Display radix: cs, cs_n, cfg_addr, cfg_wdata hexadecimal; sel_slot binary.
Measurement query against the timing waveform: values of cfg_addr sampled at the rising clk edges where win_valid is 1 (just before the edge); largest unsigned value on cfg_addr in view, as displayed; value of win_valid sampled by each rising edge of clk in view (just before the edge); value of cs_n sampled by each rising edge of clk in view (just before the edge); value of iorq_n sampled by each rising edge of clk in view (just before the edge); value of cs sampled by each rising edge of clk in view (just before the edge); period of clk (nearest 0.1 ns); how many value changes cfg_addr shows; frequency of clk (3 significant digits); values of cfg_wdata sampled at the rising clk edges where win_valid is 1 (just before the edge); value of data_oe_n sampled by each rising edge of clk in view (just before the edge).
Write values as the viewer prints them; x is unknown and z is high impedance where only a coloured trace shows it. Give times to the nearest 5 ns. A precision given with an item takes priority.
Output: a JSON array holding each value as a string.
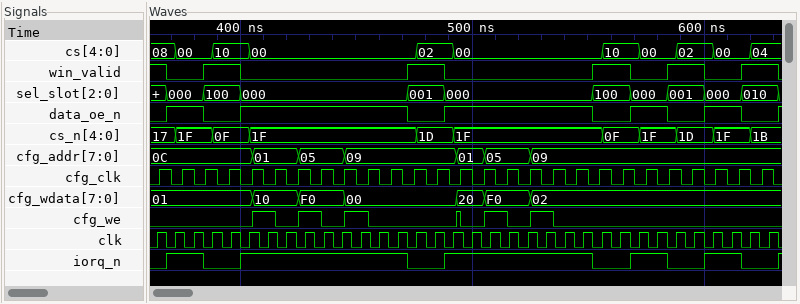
["0C, 0C, 0C, 09, 09, 09, 09, 09, 09, 09, 09", "0C", "1 0 0 1 1 0 0 0 0 0 0 0 0 0 1 1 0 0 0 0 0 0 0 0 1 1 0 0 1 1 0 0 1 1", "17, 17, 1F, 1F, 0F, 0F, 1F, 1F, 1F, 1F, 1F, 1F, 1F, 1F, 1F, 1D, 1D, 1F, 1F, 1F, 1F, 1F, 1F, 1F, 1F, 0F, 0F, 1F, 1F, 1D, 1D, 1F, 1F, 1B", "0 1 1 0 0 1 1 1 1 1 1 1 1 1 0 0 1 1 1 1 1 1 1 1 0 0 1 1 0 0 1 1 0 0", "08, 08, 00, 00, 10, 10, 00, 00, 00, 00, 00, 00, 00, 00, 00, 02, 02, 00, 00, 00, 00, 00, 00, 00, 00, 10, 10, 00, 00, 02, 02, 00, 00, 04", "8 ns", "6", "125 MHz", "01, 01, 01, 00, 00, 02, 02, 02, 02, 02, 02", "0 1 1 0 0 1 1 1 1 1 1 1 1 1 0 0 1 1 1 1 1 1 1 1 0 0 1 1 0 0 1 1 0 0"]
